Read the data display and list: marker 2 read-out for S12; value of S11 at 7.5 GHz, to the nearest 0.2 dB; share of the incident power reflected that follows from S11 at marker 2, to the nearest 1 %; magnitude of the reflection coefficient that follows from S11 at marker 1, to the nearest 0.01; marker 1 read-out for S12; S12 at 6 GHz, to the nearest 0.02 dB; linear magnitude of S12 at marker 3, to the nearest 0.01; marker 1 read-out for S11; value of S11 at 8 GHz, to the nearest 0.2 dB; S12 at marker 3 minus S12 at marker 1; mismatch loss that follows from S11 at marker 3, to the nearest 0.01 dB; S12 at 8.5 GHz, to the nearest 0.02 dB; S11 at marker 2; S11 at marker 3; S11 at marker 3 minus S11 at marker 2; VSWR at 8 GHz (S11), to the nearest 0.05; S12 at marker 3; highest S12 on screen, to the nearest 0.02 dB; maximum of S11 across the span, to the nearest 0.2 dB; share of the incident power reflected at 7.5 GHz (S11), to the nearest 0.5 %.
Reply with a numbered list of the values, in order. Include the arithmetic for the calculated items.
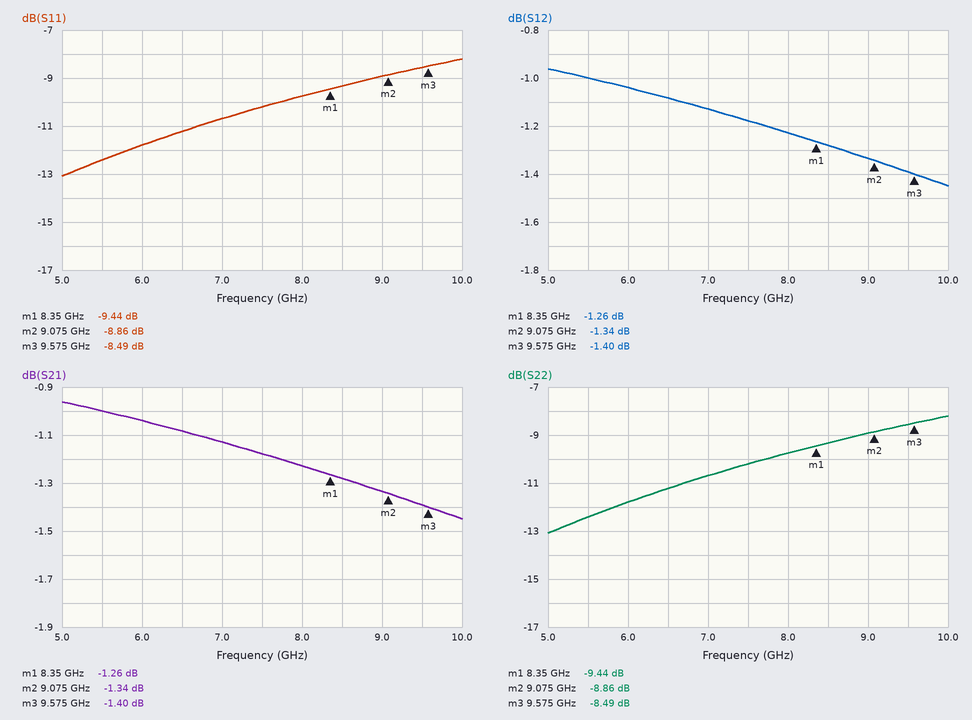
1. -1.34 dB
2. -10.2 dB
3. 10^(-8.86/10) ≈ 13 %
4. 10^(-9.44/20) ≈ 0.34
5. -1.26 dB
6. -1.04 dB
7. 10^(-1.4/20) ≈ 0.85
8. -9.44 dB
9. -9.8 dB
10. -1.4 − (-1.26) = -0.14 dB
11. −10 log10(1 − 10^(-8.49/10)) ≈ 0.66 dB
12. -1.28 dB
13. -8.86 dB
14. -8.49 dB
15. -8.49 − (-8.86) = 0.37 dB
16. |Γ| = 10^(-9.8/20) = 0.3236; VSWR = (1 + 0.3236)/(1 − 0.3236) ≈ 1.96, so 1.95 to the nearest 0.05
17. -1.40 dB
18. -0.96 dB
19. -8.2 dB
20. 10^(-10.2/10) ≈ 9.5 %
